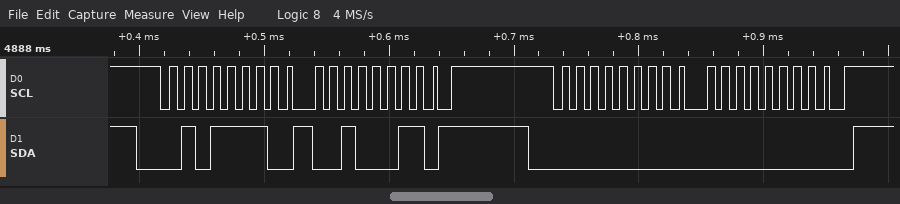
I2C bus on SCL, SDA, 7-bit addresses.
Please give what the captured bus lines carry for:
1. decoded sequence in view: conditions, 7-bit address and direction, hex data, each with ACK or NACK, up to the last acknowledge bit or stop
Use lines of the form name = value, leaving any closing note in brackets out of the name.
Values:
decoded sequence in view: conditions, 7-bit address and direction, hex data, each with ACK or NACK, up to the last acknowledge bit or stop = start, address 2F write ACK, 23 ACK, repeated start, address 00 write ACK, 00 ACK, stop
